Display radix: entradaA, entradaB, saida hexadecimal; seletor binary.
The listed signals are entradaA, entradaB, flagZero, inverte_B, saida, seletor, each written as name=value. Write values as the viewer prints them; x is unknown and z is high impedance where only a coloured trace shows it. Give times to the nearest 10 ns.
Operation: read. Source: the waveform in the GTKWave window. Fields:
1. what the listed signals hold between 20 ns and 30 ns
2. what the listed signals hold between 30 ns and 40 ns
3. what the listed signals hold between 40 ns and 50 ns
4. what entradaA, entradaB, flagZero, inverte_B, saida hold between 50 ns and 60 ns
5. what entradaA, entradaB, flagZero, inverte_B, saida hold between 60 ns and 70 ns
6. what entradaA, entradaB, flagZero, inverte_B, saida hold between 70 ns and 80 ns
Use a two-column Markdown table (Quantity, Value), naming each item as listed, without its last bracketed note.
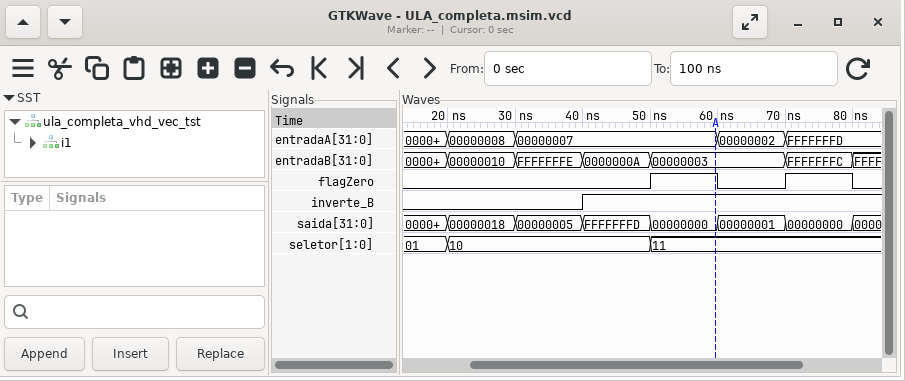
| Quantity | Value |
|---|---|
| what the listed signals hold between 20 ns and 30 ns | entradaA=00000008, entradaB=00000010, flagZero=0, inverte_B=0, saida=00000018, seletor=10 |
| what the listed signals hold between 30 ns and 40 ns | entradaA=00000007, entradaB=FFFFFFFE, flagZero=0, inverte_B=0, saida=00000005, seletor=10 |
| what the listed signals hold between 40 ns and 50 ns | entradaA=00000007, entradaB=0000000A, flagZero=0, inverte_B=1, saida=FFFFFFFD, seletor=10 |
| what entradaA, entradaB, flagZero, inverte_B, saida hold between 50 ns and 60 ns | entradaA=00000007, entradaB=00000003, flagZero=1, inverte_B=1, saida=00000000 |
| what entradaA, entradaB, flagZero, inverte_B, saida hold between 60 ns and 70 ns | entradaA=00000002, entradaB=00000003, flagZero=0, inverte_B=1, saida=00000001 |
| what entradaA, entradaB, flagZero, inverte_B, saida hold between 70 ns and 80 ns | entradaA=FFFFFFFD, entradaB=FFFFFFFC, flagZero=1, inverte_B=1, saida=00000000 |
